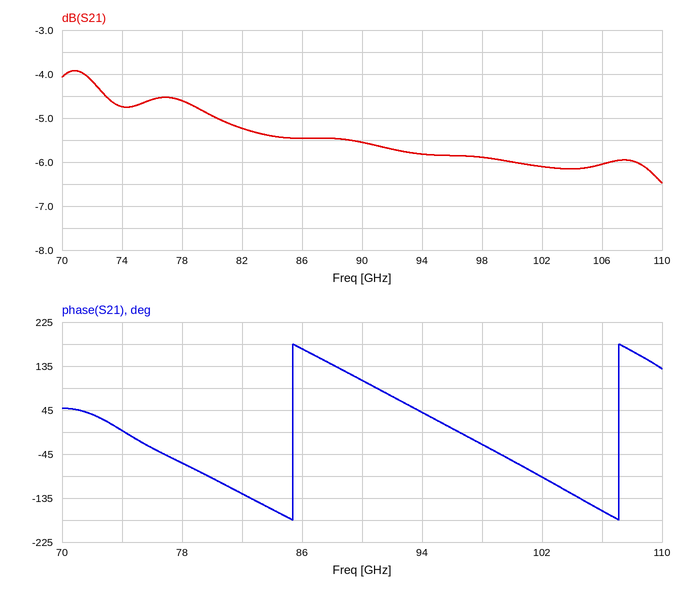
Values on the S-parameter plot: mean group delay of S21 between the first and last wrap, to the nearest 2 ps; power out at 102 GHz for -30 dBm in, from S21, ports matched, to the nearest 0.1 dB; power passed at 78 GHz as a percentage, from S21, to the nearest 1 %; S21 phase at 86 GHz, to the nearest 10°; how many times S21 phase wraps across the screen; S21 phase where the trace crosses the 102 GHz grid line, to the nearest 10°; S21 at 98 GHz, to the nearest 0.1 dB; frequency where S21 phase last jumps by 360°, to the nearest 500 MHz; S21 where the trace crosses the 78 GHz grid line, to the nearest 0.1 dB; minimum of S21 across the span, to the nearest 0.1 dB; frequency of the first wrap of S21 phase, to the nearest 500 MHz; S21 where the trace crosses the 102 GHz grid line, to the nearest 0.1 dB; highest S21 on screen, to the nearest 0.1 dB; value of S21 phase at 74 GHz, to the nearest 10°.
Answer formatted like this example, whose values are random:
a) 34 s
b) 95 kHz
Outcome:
a) 46 ps
b) -36.1 dBm
c) 35 %
d) 170°
e) 2
f) -90°
g) -5.9 dB
h) 107.0 GHz
i) -4.6 dB
j) -6.5 dB
k) 85.5 GHz
l) -6.1 dB
m) -3.9 dB
n) 0°
